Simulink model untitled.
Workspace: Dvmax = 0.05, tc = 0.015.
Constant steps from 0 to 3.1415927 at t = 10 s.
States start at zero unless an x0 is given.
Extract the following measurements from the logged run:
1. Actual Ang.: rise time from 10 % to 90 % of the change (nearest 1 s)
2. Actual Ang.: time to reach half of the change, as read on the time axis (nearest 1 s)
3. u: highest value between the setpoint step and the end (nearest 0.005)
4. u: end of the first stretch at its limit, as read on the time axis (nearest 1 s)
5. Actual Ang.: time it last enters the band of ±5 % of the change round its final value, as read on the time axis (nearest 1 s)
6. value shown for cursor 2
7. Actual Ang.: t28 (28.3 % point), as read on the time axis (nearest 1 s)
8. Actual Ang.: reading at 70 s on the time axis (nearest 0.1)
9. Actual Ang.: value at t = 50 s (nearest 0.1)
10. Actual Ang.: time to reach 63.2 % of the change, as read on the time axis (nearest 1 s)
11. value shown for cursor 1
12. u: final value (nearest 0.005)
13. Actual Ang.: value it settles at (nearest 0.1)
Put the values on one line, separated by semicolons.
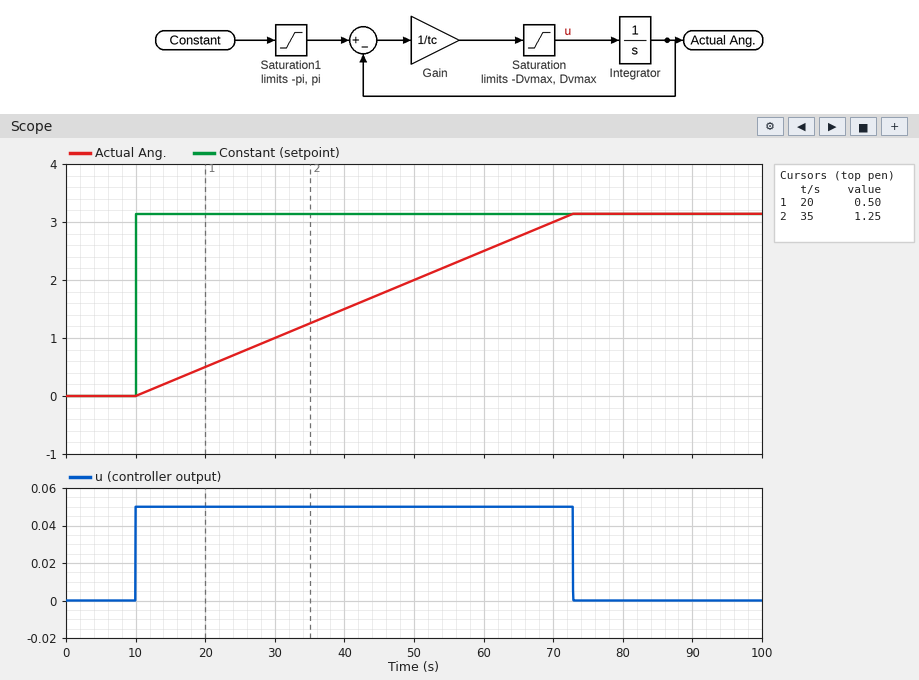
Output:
50 s; 41 s; 0.050; 73 s; 70 s; 1.25; 28 s; 3.0; 2.0; 50 s; 0.50; 0.000; 3.1
